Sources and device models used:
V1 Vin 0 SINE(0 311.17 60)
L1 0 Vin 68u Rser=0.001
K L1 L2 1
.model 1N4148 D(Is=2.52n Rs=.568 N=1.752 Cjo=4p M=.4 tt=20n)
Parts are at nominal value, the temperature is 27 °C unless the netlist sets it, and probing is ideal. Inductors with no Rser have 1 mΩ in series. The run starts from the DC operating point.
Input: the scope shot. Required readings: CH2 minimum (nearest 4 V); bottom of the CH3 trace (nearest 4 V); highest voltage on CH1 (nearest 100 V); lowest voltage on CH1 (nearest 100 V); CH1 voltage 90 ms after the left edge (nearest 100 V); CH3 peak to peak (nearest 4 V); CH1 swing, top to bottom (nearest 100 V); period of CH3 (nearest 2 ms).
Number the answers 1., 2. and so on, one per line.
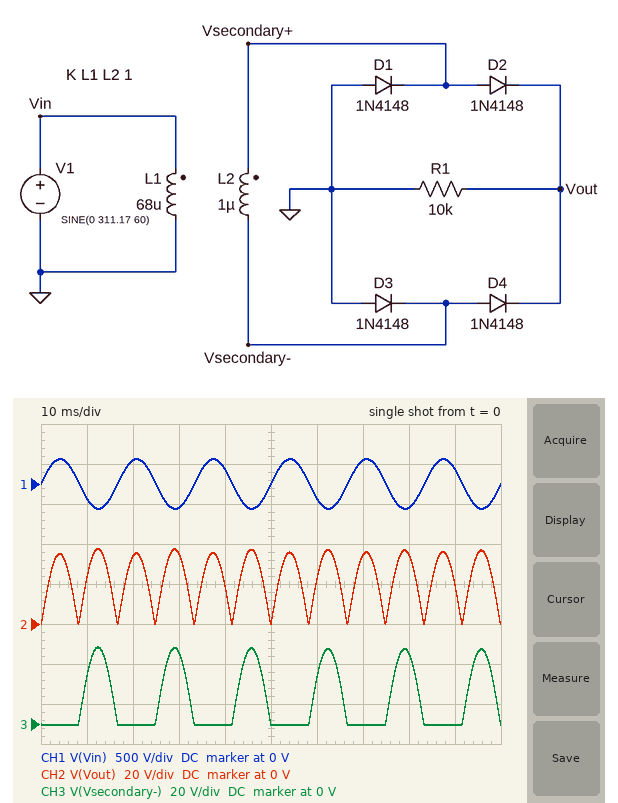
1. 0 V
2. 0 V
3. 300 V
4. -300 V
5. 200 V
6. 40 V
7. 600 V
8. 16 ms
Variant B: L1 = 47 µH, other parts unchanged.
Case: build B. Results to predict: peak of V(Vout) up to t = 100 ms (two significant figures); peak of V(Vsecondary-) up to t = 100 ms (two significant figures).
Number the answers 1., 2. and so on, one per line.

1. 46 V
2. 47 V
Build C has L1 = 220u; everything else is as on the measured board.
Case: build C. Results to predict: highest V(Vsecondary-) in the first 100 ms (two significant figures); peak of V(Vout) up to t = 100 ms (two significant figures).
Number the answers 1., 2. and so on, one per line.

1. 21 V
2. 20 V
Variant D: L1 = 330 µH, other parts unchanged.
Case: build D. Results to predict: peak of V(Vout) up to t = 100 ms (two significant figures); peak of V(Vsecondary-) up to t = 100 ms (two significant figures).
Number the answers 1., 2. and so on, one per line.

1. 16 V
2. 17 V
